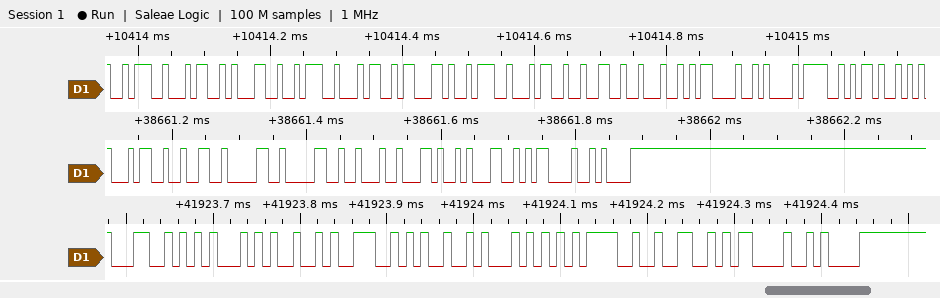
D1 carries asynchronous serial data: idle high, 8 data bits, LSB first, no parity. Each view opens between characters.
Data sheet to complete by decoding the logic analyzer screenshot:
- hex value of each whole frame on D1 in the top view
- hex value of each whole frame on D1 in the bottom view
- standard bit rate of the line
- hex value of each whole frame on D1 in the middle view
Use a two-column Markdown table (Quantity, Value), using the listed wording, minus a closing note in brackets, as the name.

| Quantity | Value |
|---|---|
| hex value of each whole frame on D1 in the top view | 3A, 34, 31, 3A, 34, 63, 3A, 34, 32, 22, 0D, 0A, 4F, 4B |
| hex value of each whole frame on D1 in the bottom view | 4C, 45, 49, 4E, 49, 54, 3D, 32, 0D, 0A |
| standard bit rate of the line | 115200 baud |
| hex value of each whole frame on D1 in the middle view | 34, 32, 30, 30, 22, 2C, 31, 0D, 0A |
